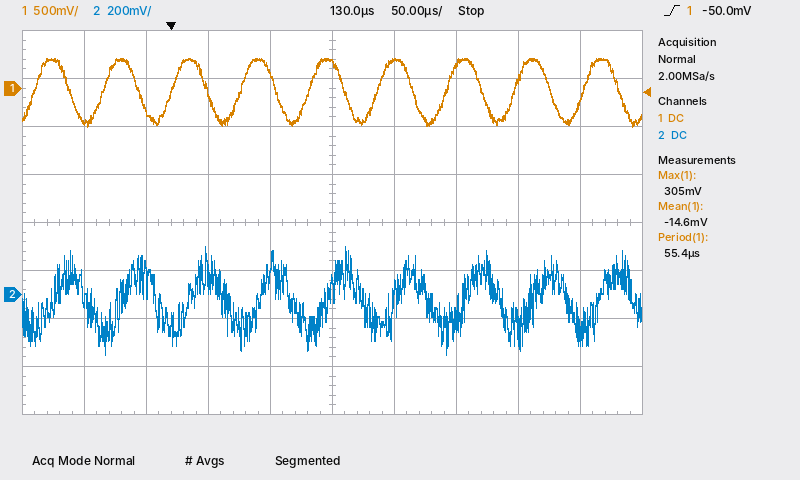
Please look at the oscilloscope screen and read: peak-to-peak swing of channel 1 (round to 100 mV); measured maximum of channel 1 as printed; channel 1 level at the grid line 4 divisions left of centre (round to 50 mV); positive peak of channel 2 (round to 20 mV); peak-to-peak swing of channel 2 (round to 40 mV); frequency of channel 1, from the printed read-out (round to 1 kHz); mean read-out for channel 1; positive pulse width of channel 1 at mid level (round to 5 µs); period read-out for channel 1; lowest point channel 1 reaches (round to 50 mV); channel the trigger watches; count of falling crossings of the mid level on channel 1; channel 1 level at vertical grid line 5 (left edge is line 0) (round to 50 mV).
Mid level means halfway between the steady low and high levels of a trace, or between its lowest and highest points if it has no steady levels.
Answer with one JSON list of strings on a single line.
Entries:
["700 mV", "305 mV", "-350 mV", "200 mV", "440 mV", "18 kHz", "-14.6 mV", "30 µs", "55.4 µs", "-400 mV", "channel 1", "9", "250 mV"]
